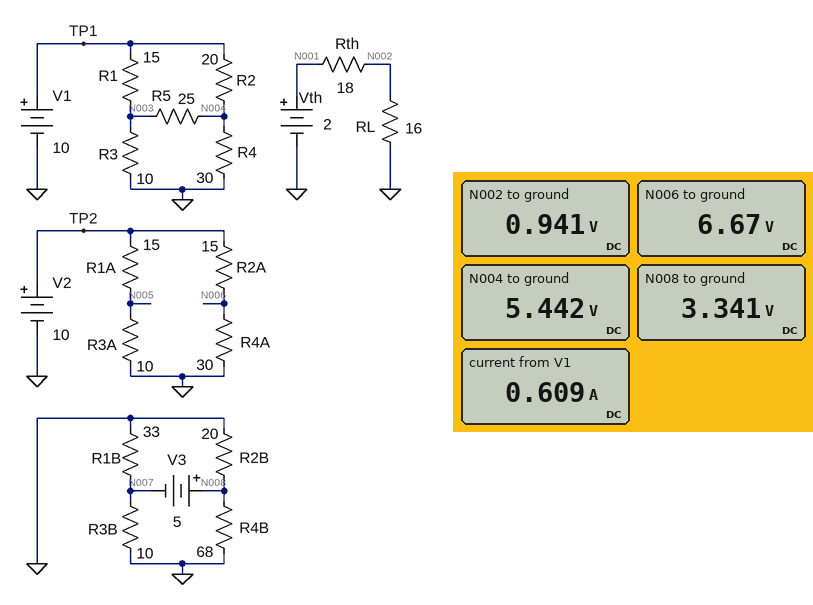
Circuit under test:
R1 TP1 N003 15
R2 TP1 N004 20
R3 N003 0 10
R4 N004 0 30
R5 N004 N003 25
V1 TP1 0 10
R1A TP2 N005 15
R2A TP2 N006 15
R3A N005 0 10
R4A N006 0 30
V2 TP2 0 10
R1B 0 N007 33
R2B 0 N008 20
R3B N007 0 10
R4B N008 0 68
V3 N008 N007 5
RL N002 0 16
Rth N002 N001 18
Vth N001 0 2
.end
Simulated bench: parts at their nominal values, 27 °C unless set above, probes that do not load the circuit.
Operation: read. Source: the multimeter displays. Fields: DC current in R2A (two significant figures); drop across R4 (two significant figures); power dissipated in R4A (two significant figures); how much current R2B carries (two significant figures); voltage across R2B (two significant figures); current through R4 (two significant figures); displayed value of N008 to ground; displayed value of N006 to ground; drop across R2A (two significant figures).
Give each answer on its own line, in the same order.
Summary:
220 mA
5.4 V
1.5 W
170 mA
3.3 V
180 mA
3.341 V
6.67 V
3.3 V
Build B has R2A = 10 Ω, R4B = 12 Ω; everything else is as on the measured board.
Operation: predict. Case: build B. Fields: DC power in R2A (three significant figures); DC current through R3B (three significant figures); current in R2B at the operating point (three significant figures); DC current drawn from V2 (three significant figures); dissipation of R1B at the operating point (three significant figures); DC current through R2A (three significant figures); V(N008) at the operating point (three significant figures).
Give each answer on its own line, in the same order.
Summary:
625 mW
253 mA
124 mA
650 mA
194 mW
250 mA
2.47 V
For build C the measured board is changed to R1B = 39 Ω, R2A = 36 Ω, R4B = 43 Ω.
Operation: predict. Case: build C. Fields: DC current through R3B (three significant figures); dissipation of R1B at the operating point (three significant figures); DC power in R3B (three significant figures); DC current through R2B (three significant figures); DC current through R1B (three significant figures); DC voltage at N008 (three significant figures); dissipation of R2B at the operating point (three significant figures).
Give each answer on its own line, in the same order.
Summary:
184 mA
87.0 mW
339 mW
158 mA
47.2 mA
3.16 V
499 mW
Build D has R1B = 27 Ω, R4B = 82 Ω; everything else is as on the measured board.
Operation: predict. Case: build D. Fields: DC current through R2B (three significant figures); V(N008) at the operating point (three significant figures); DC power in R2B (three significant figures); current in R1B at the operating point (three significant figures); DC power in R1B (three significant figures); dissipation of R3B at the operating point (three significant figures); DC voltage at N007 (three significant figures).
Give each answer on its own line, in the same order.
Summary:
172 mA
3.44 V
591 mW
57.8 mA
90.2 mW
244 mW
-1.56 V
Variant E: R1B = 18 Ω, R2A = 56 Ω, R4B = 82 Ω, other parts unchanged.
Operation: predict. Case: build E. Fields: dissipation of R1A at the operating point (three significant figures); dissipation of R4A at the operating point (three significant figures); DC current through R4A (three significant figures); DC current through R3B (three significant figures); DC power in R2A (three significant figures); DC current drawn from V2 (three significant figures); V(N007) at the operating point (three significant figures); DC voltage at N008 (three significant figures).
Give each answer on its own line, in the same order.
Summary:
2.40 W
406 mW
116 mA
143 mA
757 mW
516 mA
-1.43 V
3.57 V
